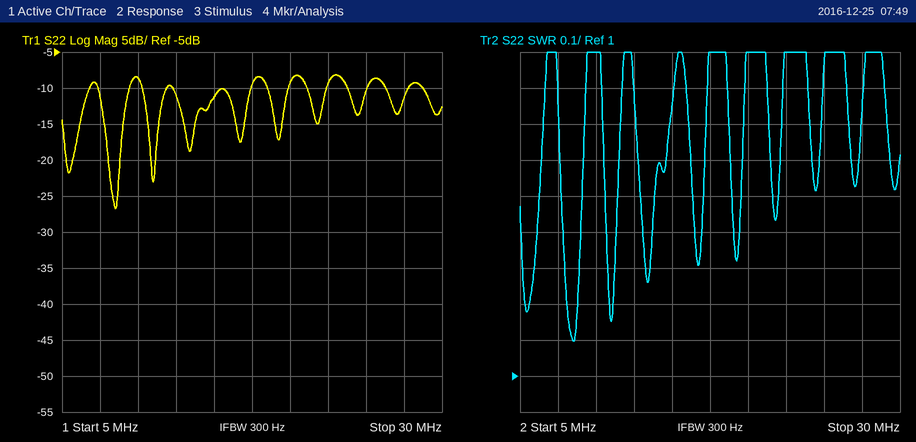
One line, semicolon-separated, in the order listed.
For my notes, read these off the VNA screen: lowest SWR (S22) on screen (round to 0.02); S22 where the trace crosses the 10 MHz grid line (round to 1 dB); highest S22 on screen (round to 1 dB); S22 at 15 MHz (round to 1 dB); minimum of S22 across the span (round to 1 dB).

1.10; -9 dB; -8 dB; -11 dB; -27 dB
